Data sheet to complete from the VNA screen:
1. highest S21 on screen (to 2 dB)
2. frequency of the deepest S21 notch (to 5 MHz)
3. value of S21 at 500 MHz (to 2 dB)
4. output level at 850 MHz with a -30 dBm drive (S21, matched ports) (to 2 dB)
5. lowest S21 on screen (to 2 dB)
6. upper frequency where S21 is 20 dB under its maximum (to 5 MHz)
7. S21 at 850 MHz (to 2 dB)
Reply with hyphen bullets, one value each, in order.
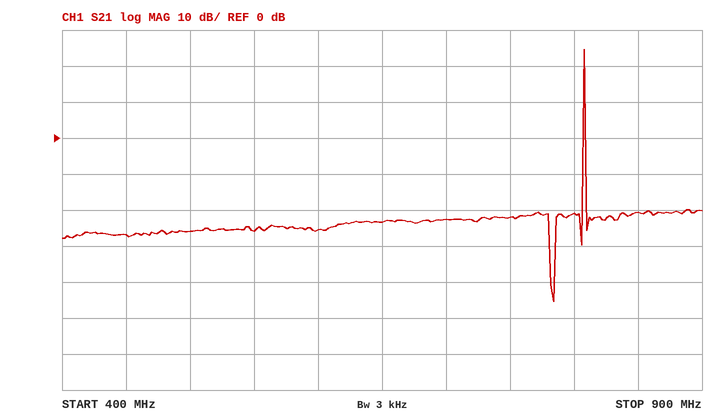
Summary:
- 24 dB
- 785 MHz
- -26 dB
- -50 dBm
- -46 dB
- 810 MHz
- -20 dB
